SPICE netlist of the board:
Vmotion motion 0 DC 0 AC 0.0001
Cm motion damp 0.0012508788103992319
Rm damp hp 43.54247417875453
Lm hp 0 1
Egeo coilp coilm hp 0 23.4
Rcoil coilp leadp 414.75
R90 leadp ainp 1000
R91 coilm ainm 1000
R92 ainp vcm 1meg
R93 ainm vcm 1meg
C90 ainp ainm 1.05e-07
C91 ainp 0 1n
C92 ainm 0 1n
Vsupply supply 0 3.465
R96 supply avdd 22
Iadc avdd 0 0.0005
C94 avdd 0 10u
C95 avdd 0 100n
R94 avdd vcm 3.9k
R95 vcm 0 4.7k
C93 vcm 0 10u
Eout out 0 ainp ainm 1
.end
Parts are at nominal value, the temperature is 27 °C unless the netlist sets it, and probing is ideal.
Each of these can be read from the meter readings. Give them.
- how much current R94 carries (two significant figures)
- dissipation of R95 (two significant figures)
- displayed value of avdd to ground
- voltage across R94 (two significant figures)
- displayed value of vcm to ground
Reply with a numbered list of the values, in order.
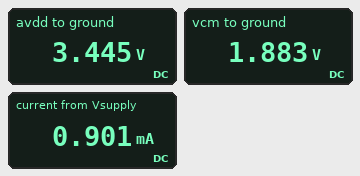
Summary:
1. 400 µA
2. 750 µW
3. 3.445 V
4. 1.6 V
5. 1.883 V
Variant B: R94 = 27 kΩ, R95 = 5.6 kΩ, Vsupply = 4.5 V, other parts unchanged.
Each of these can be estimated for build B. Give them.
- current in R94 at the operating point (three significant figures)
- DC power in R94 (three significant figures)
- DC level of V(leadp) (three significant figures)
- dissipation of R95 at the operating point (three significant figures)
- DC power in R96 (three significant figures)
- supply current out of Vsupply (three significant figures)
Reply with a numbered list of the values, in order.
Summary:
1. 138 µA
2. 511 µW
3. 771 mV
4. 106 µW
5. 8.94 µW
6. 638 µA
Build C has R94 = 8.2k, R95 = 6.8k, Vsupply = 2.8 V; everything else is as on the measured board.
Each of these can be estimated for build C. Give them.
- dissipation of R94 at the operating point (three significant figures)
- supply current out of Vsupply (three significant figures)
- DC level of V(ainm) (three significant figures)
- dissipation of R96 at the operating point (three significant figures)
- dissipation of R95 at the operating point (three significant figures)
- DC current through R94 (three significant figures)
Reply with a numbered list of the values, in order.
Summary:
1. 283 µW
2. 686 µA
3. 1.26 V
4. 10.3 µW
5. 234 µW
6. 186 µA
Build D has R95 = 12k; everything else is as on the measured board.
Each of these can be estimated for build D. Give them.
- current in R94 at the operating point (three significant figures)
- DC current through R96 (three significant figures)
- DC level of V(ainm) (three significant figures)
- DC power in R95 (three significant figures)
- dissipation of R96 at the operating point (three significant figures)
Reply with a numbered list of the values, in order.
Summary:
1. 217 µA
2. 717 µA
3. 2.60 V
4. 565 µW
5. 11.3 µW
